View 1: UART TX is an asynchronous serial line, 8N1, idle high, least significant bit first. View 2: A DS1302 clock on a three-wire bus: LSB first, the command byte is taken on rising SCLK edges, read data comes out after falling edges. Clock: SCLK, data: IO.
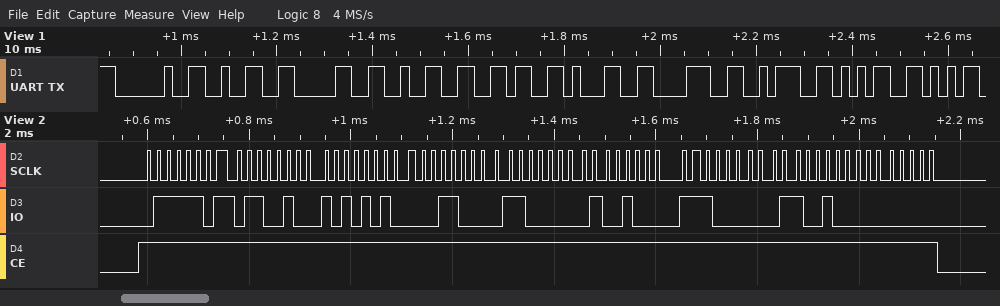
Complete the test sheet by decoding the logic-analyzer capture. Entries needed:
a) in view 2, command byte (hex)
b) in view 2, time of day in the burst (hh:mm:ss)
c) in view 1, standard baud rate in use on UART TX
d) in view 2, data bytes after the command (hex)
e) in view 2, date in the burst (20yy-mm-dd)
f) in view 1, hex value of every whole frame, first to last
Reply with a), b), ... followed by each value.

a) 0xBE
b) 18:55:26
c) 57600 baud
d) 26 55 18 06 12 07 26 00
e) 2026-12-06
f) 20 32 30 32 36 31 38 3A 35
